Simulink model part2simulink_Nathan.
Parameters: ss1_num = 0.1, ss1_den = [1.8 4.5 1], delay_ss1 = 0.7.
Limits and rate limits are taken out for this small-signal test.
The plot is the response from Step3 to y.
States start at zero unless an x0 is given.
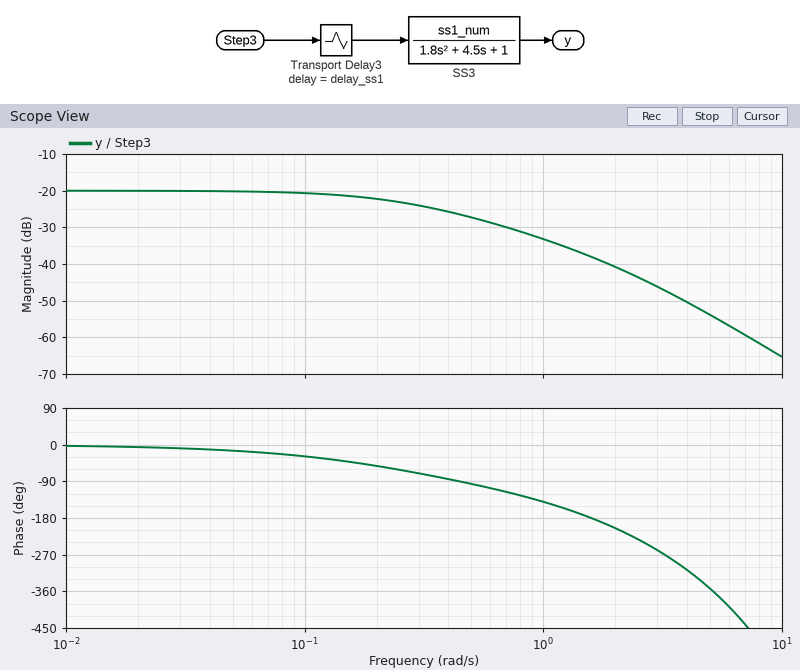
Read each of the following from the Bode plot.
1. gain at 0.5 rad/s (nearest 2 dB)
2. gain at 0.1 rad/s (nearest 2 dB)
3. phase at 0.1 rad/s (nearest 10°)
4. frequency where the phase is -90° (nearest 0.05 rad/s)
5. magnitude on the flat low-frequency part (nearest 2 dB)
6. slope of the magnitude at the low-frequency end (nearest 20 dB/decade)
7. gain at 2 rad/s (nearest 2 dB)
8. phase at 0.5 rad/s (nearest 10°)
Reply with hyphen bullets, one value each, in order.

- -28 dB
- -20 dB
- -30°
- 0.45 rad/s
- -20 dB
- 0 dB/decade
- -40 dB
- -100°
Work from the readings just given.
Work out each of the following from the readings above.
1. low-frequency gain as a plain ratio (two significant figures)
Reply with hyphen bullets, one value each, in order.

- 0.10
